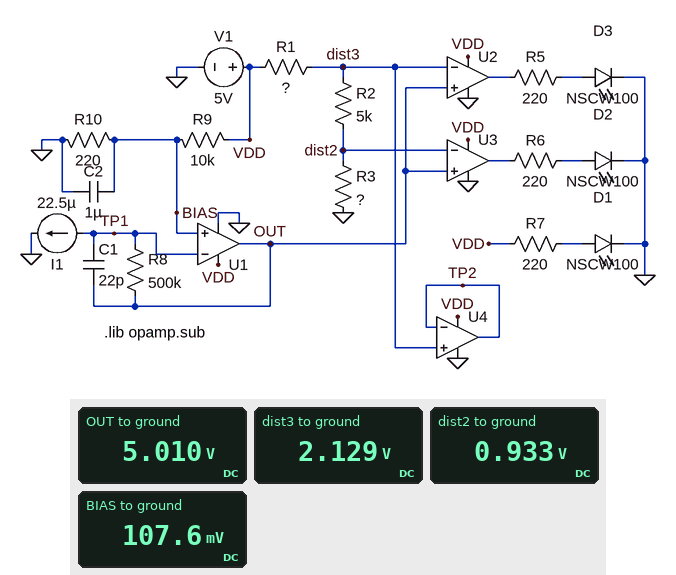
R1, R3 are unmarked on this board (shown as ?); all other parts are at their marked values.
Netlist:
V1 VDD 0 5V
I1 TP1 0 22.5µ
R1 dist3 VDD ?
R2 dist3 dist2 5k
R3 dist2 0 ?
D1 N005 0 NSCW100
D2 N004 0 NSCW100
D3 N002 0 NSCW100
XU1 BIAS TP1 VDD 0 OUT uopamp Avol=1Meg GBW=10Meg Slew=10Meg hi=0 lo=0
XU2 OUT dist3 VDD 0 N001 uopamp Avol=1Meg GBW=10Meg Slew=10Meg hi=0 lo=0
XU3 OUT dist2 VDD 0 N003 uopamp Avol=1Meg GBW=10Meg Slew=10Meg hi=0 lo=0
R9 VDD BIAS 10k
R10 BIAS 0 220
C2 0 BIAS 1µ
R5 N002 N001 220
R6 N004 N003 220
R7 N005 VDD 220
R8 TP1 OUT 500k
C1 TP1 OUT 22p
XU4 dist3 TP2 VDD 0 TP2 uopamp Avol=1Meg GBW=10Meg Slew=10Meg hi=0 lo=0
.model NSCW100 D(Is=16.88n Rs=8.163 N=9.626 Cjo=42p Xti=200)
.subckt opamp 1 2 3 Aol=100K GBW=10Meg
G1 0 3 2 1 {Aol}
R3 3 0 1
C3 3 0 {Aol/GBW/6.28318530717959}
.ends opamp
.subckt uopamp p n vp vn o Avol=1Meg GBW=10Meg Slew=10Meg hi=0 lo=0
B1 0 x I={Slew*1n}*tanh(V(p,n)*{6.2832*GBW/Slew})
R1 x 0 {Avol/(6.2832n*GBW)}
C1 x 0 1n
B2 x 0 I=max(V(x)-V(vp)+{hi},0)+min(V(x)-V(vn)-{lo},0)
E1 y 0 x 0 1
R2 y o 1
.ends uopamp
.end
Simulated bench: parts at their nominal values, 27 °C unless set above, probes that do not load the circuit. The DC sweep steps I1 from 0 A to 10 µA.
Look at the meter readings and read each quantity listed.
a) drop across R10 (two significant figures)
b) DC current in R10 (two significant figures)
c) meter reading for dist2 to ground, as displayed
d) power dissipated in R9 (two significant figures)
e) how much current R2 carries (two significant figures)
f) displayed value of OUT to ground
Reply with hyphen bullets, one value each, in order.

- 110 mV
- 490 µA
- 0.933 V
- 2.4 mW
- 240 µA
- 5.010 V
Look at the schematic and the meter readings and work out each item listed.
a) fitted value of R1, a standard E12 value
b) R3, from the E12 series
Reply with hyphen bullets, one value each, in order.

- 12 kΩ
- 3.9 kΩ
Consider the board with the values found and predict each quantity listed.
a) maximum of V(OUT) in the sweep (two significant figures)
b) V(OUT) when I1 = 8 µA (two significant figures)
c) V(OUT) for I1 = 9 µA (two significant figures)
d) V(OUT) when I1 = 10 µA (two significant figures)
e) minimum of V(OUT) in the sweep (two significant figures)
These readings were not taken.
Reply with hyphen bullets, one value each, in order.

- 5.0 V
- 4.1 V
- 4.6 V
- 5.0 V
- 110 mV
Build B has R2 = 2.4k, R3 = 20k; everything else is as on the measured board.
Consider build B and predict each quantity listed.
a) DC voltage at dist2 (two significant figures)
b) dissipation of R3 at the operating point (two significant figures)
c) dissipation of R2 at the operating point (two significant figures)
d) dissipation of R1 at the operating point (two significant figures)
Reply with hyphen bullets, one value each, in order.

- 2.9 V
- 420 µW
- 51 µW
- 250 µW
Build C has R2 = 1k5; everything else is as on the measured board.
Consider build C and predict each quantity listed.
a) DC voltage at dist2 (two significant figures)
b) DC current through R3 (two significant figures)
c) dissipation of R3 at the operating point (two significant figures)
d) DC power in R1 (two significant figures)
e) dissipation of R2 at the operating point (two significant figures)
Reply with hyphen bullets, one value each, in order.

- 1.1 V
- 290 µA
- 320 µW
- 990 µW
- 120 µW
